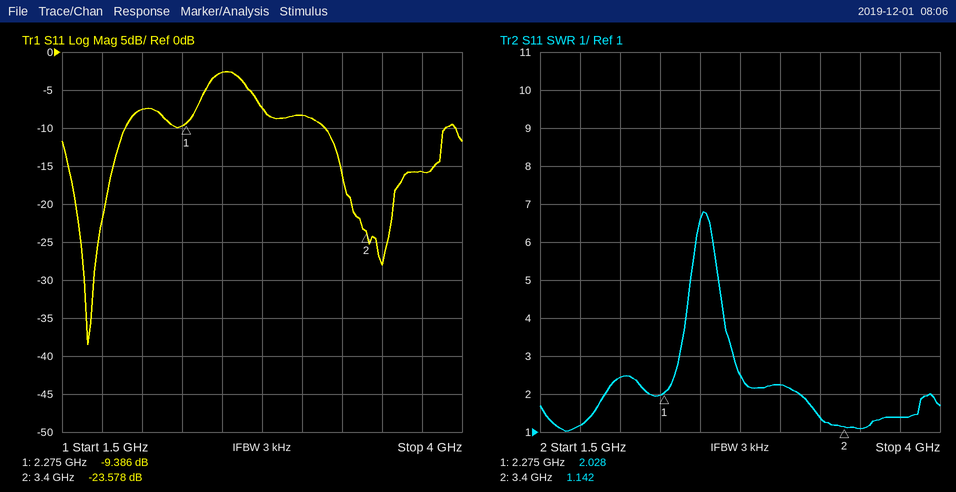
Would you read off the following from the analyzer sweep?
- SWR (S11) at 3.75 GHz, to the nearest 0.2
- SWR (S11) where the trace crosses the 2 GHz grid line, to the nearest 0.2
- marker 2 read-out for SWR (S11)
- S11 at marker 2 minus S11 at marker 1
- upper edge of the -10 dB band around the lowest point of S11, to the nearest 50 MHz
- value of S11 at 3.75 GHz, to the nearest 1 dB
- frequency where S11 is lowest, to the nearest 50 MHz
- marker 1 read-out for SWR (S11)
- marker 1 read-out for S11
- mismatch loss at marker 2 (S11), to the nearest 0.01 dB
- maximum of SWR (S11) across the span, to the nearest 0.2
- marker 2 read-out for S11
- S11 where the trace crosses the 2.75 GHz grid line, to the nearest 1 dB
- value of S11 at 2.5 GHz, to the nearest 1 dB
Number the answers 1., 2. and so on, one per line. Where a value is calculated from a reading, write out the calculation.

1. 1.4
2. 2.4
3. 1.142
4. -23.578 − (-9.386) = -14.192 dB
5. 1.90 GHz
6. -16 dB
7. 1.65 GHz
8. 2.028
9. -9.386 dB
10. −10 log10(1 − 10^(-23.578/10)) ≈ 0.02 dB
11. 6.8
12. -23.578 dB
13. -7 dB
14. -3 dB
